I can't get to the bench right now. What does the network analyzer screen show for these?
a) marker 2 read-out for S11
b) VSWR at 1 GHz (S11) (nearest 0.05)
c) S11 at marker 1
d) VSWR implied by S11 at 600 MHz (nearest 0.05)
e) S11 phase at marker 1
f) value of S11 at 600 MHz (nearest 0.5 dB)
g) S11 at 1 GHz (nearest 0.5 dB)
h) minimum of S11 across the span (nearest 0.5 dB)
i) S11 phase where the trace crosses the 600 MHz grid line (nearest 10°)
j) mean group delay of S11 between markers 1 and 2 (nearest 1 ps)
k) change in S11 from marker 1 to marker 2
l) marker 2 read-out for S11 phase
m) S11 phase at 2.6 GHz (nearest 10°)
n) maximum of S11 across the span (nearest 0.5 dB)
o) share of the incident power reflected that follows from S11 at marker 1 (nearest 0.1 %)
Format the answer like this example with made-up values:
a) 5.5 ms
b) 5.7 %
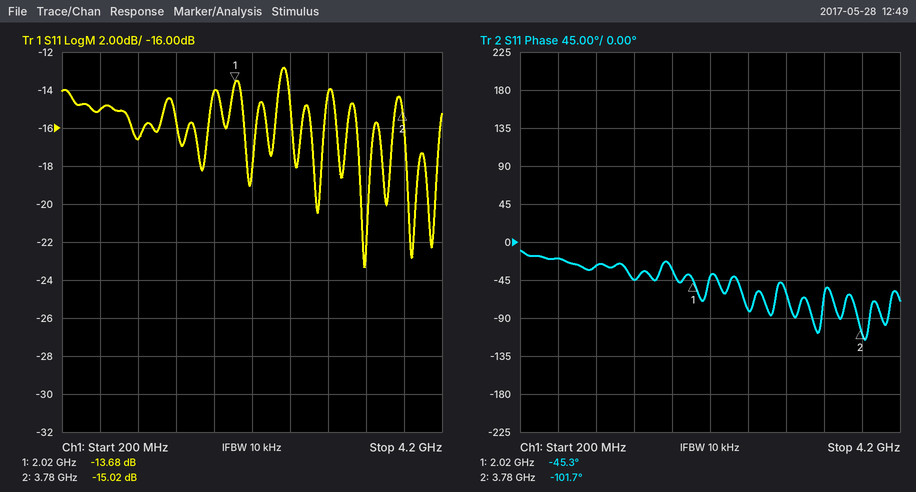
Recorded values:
a) -15.02 dB
b) 1.35
c) -13.68 dB
d) 1.45
e) -45.3°
f) -15.0 dB
g) -16.5 dB
h) -23.5 dB
i) -20°
j) 89 ps
k) -1.34 dB
l) -101.7°
m) -80°
n) -13.0 dB
o) 4.3 %
